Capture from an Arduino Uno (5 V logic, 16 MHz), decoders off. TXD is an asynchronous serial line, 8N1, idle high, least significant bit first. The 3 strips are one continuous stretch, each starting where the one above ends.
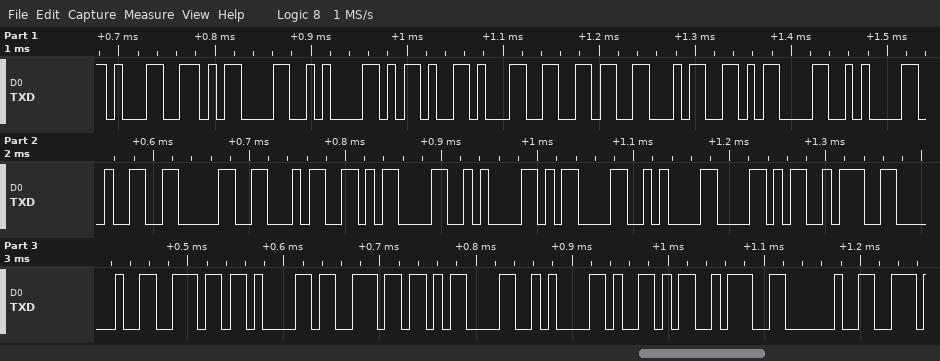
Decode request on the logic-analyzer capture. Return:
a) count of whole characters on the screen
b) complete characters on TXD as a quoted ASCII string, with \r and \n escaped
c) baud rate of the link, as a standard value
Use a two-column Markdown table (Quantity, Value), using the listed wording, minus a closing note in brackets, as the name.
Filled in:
| Quantity | Value |
|---|---|
| count of whole characters on the screen | 27 |
| complete characters on TXD as a quoted ASCII string, with \r and \n escaped | "1\r\n-164\r\n204\r\n\r\nX: nan\r\nY: " |
| baud rate of the link, as a standard value | 115200 baud |
